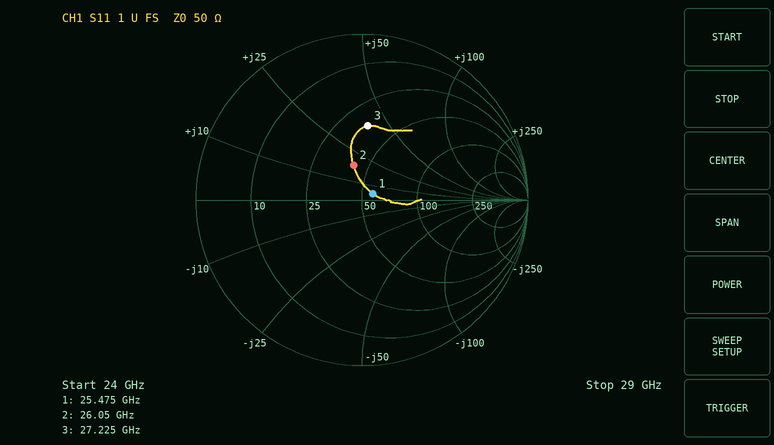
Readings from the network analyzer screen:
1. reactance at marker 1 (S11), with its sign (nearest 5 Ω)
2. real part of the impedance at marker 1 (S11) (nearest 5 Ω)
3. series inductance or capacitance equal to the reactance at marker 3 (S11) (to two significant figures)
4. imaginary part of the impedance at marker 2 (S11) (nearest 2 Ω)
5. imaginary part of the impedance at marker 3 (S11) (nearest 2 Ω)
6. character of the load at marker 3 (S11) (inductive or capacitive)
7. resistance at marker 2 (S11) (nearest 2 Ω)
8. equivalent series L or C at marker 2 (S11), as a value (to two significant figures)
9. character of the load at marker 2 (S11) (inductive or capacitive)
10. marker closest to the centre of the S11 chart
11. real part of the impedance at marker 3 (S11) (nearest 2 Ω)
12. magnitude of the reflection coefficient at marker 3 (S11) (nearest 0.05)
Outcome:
+5 Ω
55 Ω
230 pH
+18 Ω
+40 Ω
inductive
42 Ω
110 pH
inductive
marker 1
36 Ω
0.45
